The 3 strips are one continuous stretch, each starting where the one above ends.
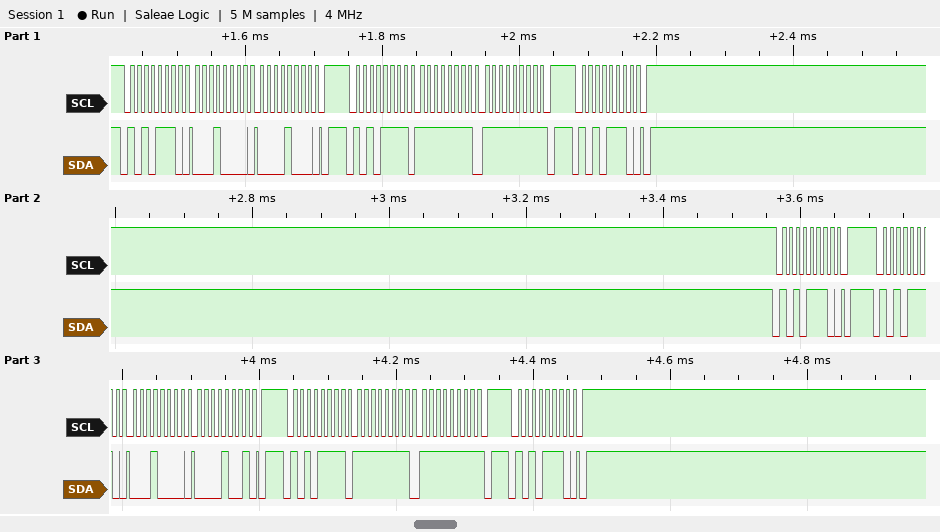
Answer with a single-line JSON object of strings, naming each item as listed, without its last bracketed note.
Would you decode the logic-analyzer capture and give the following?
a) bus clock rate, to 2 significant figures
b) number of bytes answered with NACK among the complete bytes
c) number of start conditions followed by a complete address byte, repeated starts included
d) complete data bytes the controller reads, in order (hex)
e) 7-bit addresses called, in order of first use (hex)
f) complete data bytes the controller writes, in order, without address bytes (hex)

{"bus clock rate, to 2 significant figures": "100 kHz", "number of bytes answered with NACK among the complete bytes": "2", "number of start conditions followed by a complete address byte, repeated starts included": "7", "complete data bytes the controller reads, in order": "FF FF FF FF", "7-bit addresses called, in order of first use": "0x57", "complete data bytes the controller writes, in order, without address bytes": "10 08 10 09"}
